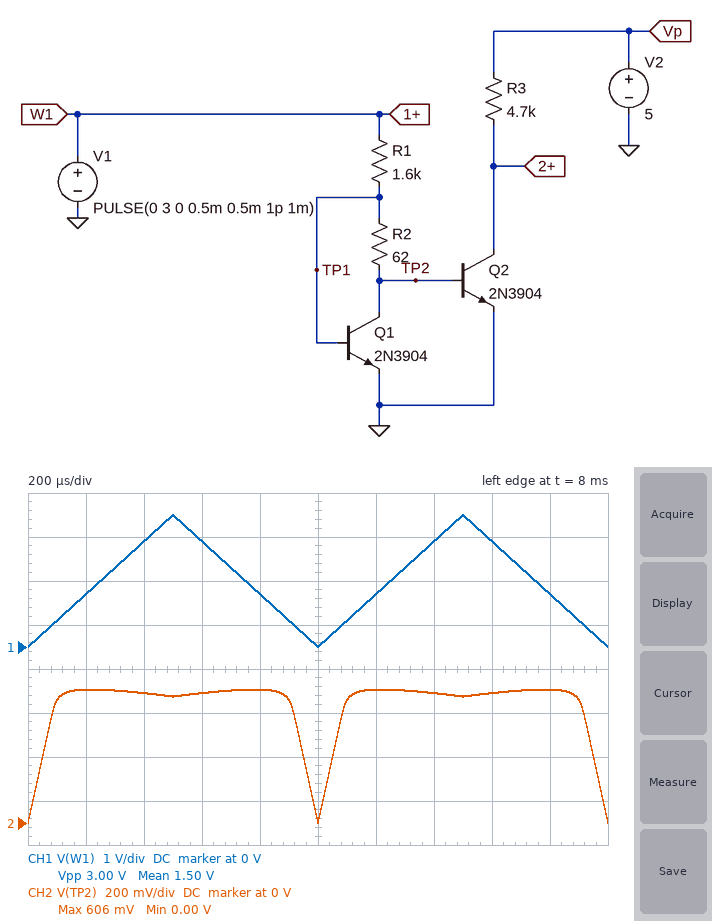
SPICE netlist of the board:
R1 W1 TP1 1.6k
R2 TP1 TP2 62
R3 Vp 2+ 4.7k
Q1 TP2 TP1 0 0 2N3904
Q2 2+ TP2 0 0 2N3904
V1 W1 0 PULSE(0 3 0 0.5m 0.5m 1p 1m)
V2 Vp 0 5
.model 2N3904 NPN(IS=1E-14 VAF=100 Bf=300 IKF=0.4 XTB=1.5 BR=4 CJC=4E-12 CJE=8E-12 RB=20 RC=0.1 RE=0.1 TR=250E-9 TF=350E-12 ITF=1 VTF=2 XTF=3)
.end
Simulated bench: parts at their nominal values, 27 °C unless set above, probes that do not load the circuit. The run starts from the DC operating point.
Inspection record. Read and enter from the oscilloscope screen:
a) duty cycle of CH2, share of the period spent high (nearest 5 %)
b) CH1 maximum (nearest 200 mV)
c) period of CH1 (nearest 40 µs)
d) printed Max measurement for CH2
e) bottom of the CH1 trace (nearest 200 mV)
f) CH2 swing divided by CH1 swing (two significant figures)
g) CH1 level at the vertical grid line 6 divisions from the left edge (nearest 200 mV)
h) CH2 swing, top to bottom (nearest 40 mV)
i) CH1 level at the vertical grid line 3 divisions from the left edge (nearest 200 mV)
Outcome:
90 %
3.0 V
1.00 ms
606 mV
0 V
0.20
1.2 V
600 mV
2.4 V
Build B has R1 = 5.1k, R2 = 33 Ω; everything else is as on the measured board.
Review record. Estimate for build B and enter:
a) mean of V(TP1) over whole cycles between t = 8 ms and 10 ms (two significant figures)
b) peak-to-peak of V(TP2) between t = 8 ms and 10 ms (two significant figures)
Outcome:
550 mV
620 mV
